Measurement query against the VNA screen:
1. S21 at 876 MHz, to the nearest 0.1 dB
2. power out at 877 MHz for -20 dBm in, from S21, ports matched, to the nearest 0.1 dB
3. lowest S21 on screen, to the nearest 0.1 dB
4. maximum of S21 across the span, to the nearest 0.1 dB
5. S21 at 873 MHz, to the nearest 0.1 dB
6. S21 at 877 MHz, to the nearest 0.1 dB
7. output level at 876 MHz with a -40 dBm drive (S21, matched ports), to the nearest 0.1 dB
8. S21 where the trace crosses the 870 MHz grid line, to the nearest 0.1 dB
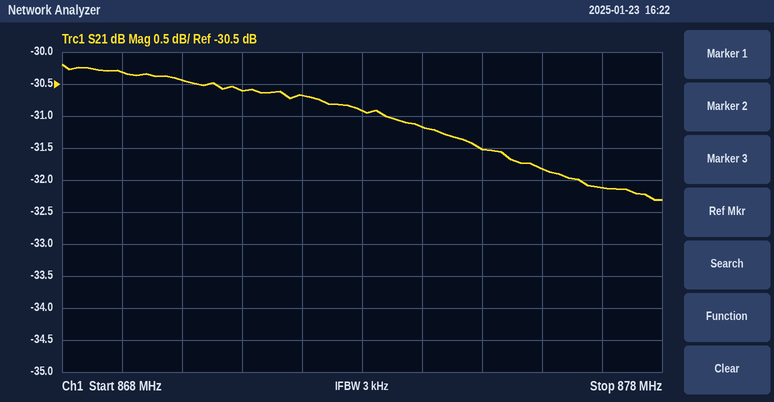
-31.8 dB
-52.1 dBm
-32.3 dB
-30.2 dB
-30.9 dB
-32.1 dB
-71.8 dBm
-30.4 dB
